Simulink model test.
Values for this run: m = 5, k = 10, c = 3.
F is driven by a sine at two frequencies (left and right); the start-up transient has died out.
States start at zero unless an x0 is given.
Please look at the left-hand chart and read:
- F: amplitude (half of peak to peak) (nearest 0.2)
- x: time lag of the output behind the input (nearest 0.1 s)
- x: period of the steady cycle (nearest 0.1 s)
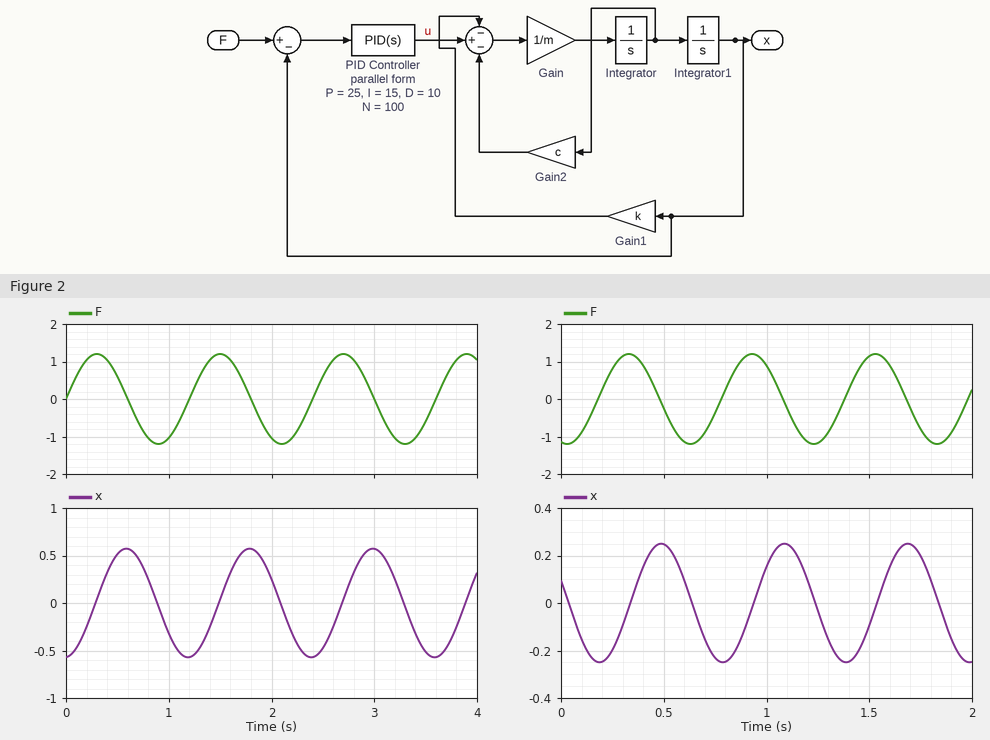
1.2
0.3 s
1.2 s
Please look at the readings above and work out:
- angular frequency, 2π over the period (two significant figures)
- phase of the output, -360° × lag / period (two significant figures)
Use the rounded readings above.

5.2 rad/s
-90°
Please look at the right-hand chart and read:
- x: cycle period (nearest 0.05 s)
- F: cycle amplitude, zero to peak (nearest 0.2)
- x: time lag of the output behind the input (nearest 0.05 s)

0.60 s
1.2
0.15 s
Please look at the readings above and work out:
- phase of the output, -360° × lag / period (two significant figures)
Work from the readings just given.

-90°
